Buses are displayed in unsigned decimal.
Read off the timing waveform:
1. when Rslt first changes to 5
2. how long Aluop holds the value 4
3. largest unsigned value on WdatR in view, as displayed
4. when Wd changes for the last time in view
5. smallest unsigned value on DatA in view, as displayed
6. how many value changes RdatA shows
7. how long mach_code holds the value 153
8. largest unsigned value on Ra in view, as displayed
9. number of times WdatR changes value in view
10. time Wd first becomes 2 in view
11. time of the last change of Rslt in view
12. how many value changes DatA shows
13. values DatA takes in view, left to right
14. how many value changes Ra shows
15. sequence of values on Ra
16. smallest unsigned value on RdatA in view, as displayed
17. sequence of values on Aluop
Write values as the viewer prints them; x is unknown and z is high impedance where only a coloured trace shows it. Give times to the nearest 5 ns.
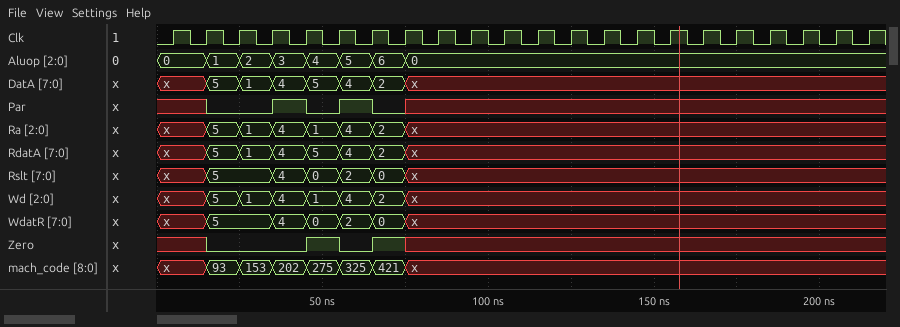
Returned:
15 ns
10 ns
5
75 ns
1
7
10 ns
5
6
65 ns
75 ns
7
x, 5, 1, 4, 5, 4, 2, x
7
x, 5, 1, 4, 1, 4, 2, x
1
0, 1, 2, 3, 4, 5, 6, 0
